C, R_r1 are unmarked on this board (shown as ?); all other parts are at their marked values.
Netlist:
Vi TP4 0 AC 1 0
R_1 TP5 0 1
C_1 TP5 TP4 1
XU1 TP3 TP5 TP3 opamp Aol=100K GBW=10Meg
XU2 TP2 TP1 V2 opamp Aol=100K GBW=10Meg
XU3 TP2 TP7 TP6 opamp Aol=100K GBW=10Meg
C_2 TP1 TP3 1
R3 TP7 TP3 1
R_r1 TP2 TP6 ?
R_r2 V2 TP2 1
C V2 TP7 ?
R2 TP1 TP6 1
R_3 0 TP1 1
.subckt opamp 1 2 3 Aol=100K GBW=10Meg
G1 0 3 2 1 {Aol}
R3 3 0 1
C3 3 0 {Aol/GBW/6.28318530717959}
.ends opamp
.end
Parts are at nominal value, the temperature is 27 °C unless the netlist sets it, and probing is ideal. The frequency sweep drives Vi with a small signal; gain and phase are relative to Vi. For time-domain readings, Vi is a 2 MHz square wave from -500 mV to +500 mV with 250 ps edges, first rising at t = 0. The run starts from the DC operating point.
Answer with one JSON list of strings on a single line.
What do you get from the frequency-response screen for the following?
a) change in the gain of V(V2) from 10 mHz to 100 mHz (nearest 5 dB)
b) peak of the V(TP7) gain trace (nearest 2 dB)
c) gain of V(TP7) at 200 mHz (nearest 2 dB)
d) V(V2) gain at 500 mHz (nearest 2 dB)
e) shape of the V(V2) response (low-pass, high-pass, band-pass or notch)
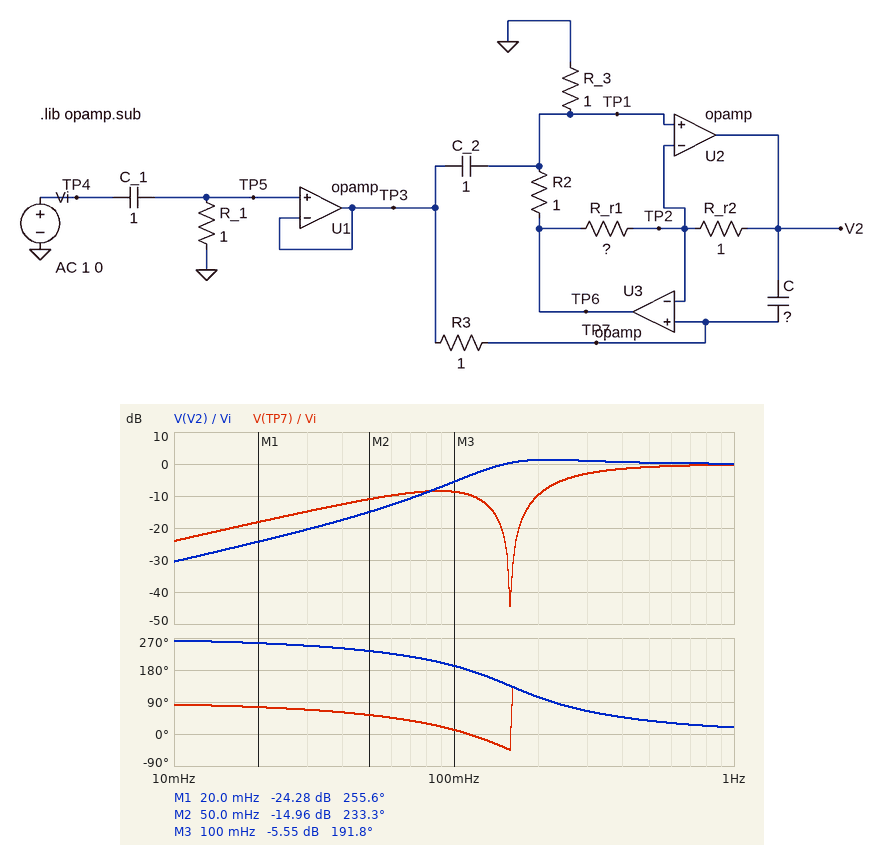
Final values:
["25 dB", "0 dB", "-10 dB", "0 dB", "high-pass"]
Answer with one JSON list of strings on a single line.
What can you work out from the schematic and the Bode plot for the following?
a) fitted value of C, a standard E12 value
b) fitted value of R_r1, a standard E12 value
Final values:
["680 mF", "0.68 Ω"]
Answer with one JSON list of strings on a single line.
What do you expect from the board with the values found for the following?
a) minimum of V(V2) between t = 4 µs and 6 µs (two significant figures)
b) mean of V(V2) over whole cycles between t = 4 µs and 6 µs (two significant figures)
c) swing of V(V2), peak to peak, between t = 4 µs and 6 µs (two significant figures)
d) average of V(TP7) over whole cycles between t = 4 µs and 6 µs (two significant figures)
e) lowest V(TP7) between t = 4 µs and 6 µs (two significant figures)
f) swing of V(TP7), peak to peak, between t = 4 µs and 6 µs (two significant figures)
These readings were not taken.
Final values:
["-150 mV", "500 mV", "1.3 V", "500 mV", "-150 mV", "1.3 V"]
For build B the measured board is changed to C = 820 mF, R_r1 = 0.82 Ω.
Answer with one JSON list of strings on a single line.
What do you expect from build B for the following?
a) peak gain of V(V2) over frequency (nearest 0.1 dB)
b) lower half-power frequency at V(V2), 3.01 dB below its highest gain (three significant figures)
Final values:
["0.5 dB", "143 mHz"]
